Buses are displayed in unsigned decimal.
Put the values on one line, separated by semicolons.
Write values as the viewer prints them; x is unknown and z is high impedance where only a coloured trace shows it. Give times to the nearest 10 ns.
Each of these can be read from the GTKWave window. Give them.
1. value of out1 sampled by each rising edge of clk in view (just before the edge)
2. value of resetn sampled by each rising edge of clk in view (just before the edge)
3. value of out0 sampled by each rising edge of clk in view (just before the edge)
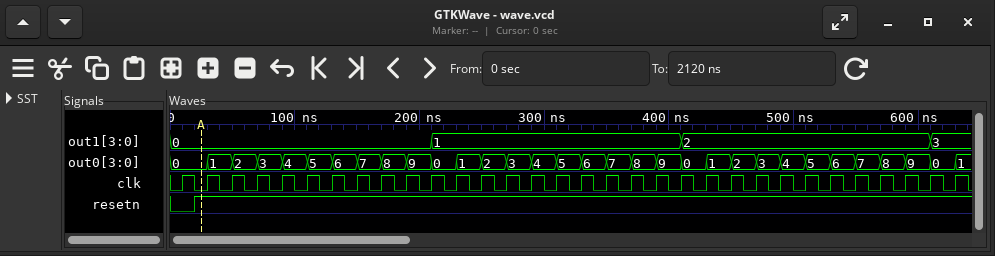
0, 0, 0, 0, 0, 0, 0, 0, 0, 0, 0, 1, 1, 1, 1, 1, 1, 1, 1, 1, 1, 2, 2, 2, 2, 2, 2, 2, 2, 2, 2, 3; 0 1 1 1 1 1 1 1 1 1 1 1 1 1 1 1 1 1 1 1 1 1 1 1 1 1 1 1 1 1 1 1; 0, 0, 1, 2, 3, 4, 5, 6, 7, 8, 9, 0, 1, 2, 3, 4, 5, 6, 7, 8, 9, 0, 1, 2, 3, 4, 5, 6, 7, 8, 9, 0
